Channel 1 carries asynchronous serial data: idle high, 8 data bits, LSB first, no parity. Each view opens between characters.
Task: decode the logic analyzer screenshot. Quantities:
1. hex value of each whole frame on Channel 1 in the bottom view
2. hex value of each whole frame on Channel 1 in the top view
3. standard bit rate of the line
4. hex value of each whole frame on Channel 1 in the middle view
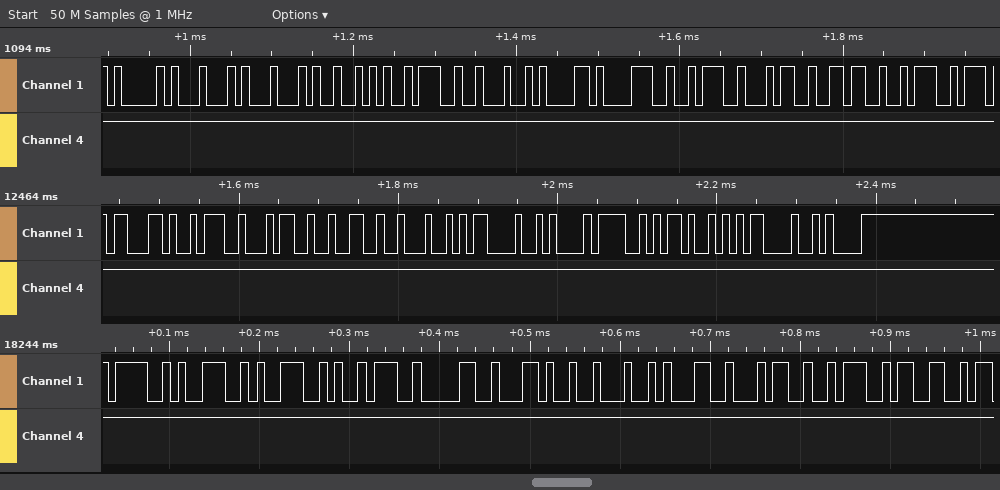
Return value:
4F, 4E, 4E, 3A, 30, 2C, 22, 31, 34, 3A, 33
41, 44, 44, 52, 3A, 22, 61, 38, 3A, 34, 36, 3A
115200 baud
63, 3A, 34, 32, 22, 0D, 0A, 4F, 4B, 0D, 0A
